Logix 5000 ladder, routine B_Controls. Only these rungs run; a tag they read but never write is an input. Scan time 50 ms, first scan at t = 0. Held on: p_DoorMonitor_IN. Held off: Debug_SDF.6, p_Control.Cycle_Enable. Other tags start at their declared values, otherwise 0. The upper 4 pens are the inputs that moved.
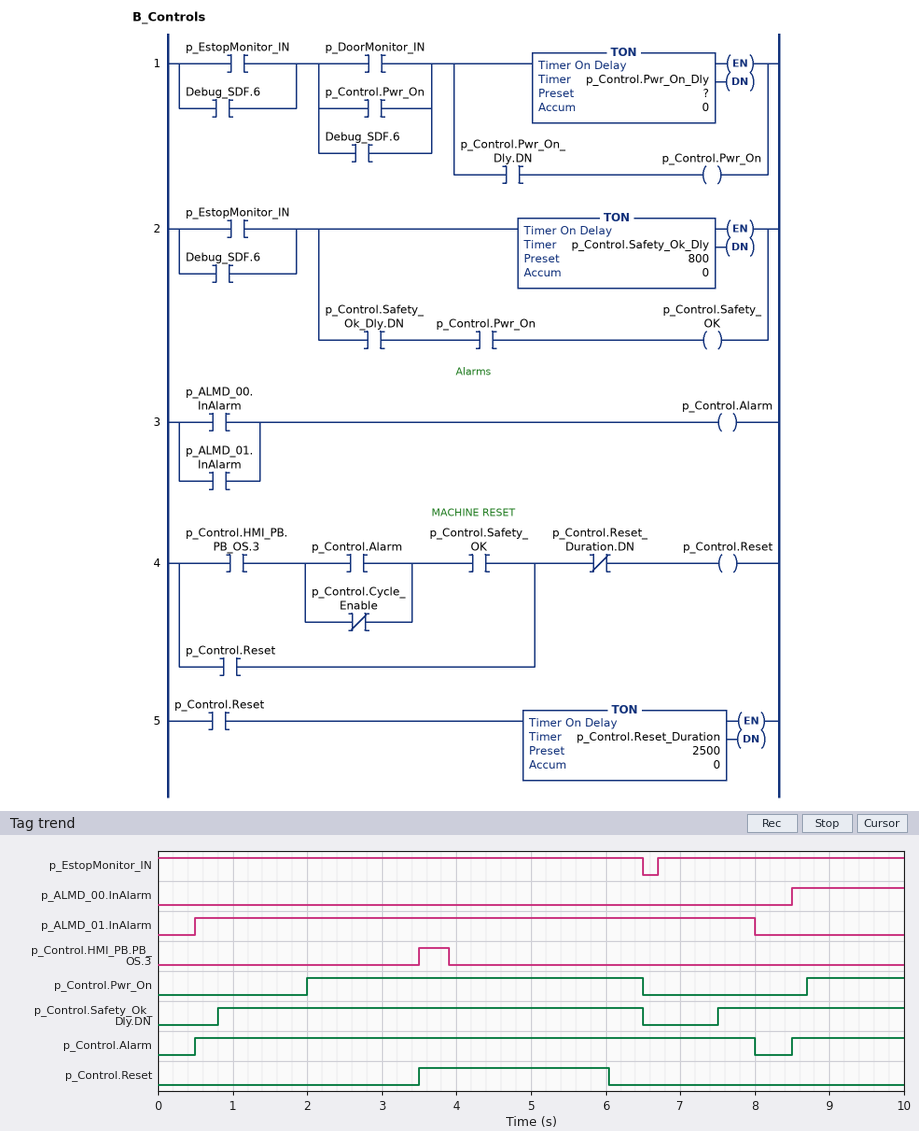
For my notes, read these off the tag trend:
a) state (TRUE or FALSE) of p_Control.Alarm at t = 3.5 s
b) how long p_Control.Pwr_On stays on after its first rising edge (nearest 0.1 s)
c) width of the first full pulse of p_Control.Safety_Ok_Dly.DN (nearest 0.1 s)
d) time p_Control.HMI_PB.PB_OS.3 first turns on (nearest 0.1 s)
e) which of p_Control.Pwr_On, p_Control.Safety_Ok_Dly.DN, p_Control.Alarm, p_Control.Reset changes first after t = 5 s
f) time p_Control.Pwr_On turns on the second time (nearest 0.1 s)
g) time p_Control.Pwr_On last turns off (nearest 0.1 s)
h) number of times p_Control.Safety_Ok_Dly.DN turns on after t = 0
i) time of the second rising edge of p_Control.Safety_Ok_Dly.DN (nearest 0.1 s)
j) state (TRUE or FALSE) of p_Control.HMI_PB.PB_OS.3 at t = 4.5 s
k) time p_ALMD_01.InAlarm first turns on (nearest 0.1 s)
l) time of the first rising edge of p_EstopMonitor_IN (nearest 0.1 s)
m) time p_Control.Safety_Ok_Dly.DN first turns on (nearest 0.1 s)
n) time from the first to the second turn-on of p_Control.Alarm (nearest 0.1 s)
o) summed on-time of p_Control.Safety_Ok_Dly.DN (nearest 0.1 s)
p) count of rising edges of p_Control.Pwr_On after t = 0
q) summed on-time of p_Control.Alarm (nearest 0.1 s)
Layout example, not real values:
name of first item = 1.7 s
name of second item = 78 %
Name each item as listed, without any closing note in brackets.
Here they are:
state (TRUE or FALSE) of p_Control.Alarm at t = 3.5 s = TRUE
how long p_Control.Pwr_On stays on after its first rising edge = 4.5 s
width of the first full pulse of p_Control.Safety_Ok_Dly.DN = 5.7 s
time p_Control.HMI_PB.PB_OS.3 first turns on = 3.5 s
which of p_Control.Pwr_On, p_Control.Safety_Ok_Dly.DN, p_Control.Alarm, p_Control.Reset changes first after t = 5 s = p_Control.Reset
time p_Control.Pwr_On turns on the second time = 8.7 s
time p_Control.Pwr_On last turns off = 6.5 s
number of times p_Control.Safety_Ok_Dly.DN turns on after t = 0 = 2
time of the second rising edge of p_Control.Safety_Ok_Dly.DN = 7.5 s
state (TRUE or FALSE) of p_Control.HMI_PB.PB_OS.3 at t = 4.5 s = FALSE
time p_ALMD_01.InAlarm first turns on = 0.5 s
time of the first rising edge of p_EstopMonitor_IN = 6.7 s
time p_Control.Safety_Ok_Dly.DN first turns on = 0.8 s
time from the first to the second turn-on of p_Control.Alarm = 8.0 s
summed on-time of p_Control.Safety_Ok_Dly.DN = 8.2 s
count of rising edges of p_Control.Pwr_On after t = 0 = 2
summed on-time of p_Control.Alarm = 9.0 s
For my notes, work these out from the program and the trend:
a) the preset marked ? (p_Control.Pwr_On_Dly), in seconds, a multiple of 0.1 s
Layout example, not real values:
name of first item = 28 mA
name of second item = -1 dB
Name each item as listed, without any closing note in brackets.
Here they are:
the preset marked ? (p_Control.Pwr_On_Dly), in seconds, a multiple of 0.1 s = 2.0 s
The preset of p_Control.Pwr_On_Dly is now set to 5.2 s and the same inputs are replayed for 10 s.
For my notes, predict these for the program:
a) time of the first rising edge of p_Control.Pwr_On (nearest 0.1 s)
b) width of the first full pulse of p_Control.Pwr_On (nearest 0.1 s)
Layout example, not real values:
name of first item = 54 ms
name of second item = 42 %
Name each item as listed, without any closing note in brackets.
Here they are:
time of the first rising edge of p_Control.Pwr_On = 5.2 s
width of the first full pulse of p_Control.Pwr_On = 1.3 s
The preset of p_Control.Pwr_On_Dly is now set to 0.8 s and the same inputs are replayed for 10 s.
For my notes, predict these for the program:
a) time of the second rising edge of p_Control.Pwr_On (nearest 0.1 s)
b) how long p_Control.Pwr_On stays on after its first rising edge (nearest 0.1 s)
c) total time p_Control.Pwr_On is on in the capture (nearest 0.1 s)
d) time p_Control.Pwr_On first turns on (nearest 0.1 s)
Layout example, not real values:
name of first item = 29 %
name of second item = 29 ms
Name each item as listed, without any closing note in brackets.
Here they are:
time of the second rising edge of p_Control.Pwr_On = 7.5 s
how long p_Control.Pwr_On stays on after its first rising edge = 5.7 s
total time p_Control.Pwr_On is on in the capture = 8.2 s
time p_Control.Pwr_On first turns on = 0.8 s
